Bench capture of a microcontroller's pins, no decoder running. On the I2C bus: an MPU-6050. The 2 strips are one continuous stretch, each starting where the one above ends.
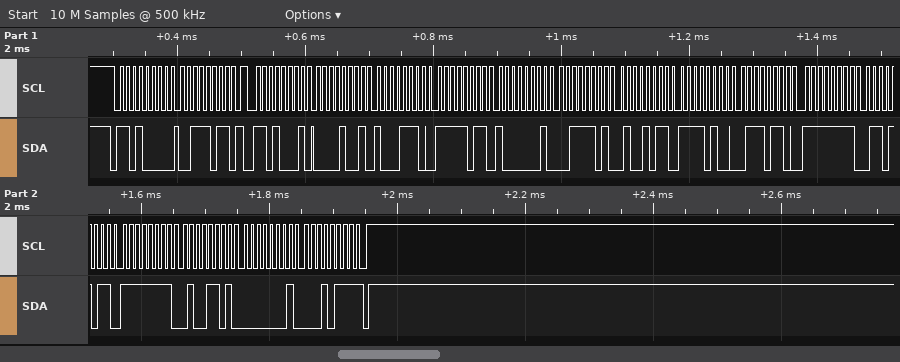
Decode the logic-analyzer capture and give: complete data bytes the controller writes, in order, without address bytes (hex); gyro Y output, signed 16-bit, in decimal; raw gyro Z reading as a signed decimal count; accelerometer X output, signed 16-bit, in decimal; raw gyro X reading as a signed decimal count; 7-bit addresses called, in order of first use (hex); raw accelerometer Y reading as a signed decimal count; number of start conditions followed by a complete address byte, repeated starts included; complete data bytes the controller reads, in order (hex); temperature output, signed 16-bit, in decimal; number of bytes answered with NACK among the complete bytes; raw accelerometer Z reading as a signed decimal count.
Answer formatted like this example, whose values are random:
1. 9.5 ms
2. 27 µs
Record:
1. 3B
2. -179
3. 279
4. 2446
5. -149
6. 0x68
7. -1151
8. 2
9. 09 8E FB 81 3D 4B F4 76 FF 6B FF 4D 01 17
10. -2954
11. 1
12. 15691
